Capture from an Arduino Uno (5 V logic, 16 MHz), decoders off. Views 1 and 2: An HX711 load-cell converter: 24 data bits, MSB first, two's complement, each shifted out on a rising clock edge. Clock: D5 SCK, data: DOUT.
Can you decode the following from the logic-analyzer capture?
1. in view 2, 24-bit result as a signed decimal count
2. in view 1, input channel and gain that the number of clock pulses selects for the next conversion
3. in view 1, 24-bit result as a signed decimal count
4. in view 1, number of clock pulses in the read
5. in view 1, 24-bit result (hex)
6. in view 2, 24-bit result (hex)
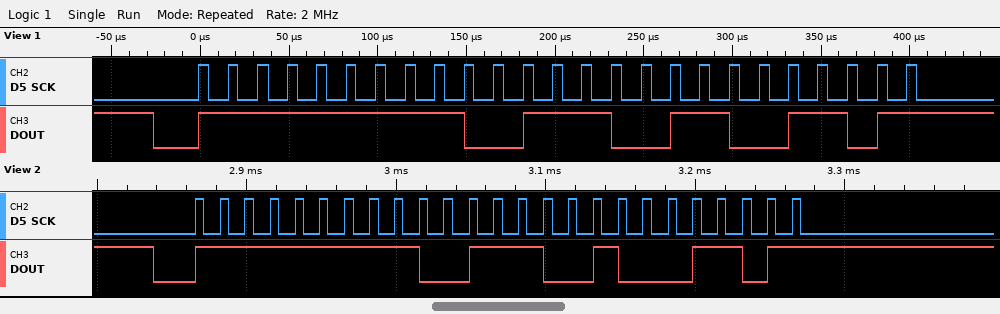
-25459
channel A, gain 128
-25395
25
0xFF9CCD
0xFF9C8D
